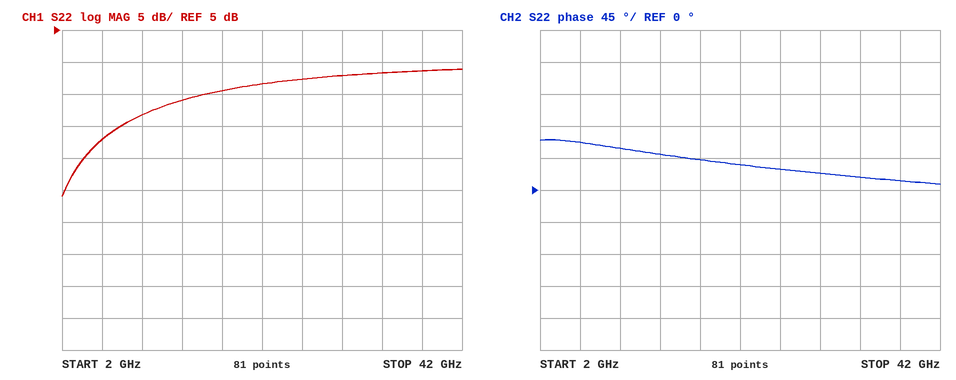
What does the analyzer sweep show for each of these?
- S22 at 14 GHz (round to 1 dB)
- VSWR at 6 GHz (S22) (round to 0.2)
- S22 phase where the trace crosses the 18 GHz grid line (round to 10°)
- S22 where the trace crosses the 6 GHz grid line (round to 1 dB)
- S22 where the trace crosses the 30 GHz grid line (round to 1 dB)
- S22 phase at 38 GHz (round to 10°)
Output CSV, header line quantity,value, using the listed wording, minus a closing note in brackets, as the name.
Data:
quantity,value
S22 at 14 GHz,-6 dB
VSWR at 6 GHz (S22),1.6
S22 phase where the trace crosses the 18 GHz grid line,40°
S22 where the trace crosses the 6 GHz grid line,-12 dB
S22 where the trace crosses the 30 GHz grid line,-2 dB
S22 phase at 38 GHz,10°
